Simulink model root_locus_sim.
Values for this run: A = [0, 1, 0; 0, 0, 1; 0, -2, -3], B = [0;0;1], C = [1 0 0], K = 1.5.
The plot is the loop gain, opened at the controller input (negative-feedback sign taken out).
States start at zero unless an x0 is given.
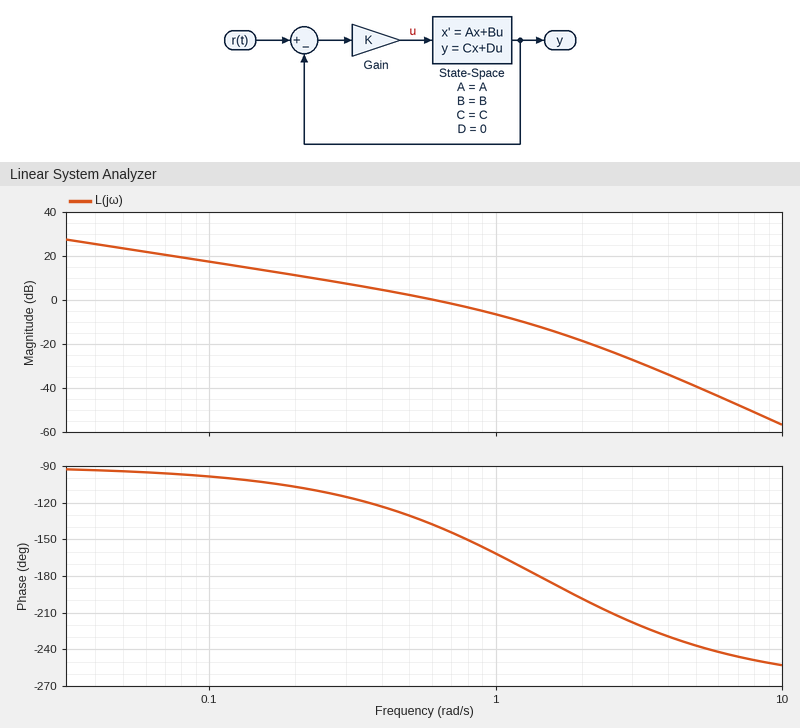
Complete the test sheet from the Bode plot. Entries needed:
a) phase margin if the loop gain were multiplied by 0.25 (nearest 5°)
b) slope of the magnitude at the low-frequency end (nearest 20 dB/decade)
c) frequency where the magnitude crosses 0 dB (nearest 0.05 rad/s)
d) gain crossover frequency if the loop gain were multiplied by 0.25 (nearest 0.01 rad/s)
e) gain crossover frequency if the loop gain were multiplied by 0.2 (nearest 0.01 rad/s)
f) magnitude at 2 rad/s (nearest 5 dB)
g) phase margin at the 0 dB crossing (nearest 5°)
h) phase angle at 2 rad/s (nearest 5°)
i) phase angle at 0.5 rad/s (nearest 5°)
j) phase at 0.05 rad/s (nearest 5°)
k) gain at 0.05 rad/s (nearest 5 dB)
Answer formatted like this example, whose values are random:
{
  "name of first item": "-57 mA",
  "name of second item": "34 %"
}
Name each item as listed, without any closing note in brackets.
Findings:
{
  "phase margin if the loop gain were multiplied by 0.25": "75°",
  "slope of the magnitude at the low-frequency end": "-20 dB/decade",
  "frequency where the magnitude crosses 0 dB": "0.60 rad/s",
  "gain crossover frequency if the loop gain were multiplied by 0.25": "0.18 rad/s",
  "gain crossover frequency if the loop gain were multiplied by 0.2": "0.15 rad/s",
  "magnitude at 2 rad/s": "-20 dB",
  "phase margin at the 0 dB crossing": "40°",
  "phase angle at 2 rad/s": "-200°",
  "phase angle at 0.5 rad/s": "-130°",
  "phase at 0.05 rad/s": "-95°",
  "gain at 0.05 rad/s": "25 dB"
}
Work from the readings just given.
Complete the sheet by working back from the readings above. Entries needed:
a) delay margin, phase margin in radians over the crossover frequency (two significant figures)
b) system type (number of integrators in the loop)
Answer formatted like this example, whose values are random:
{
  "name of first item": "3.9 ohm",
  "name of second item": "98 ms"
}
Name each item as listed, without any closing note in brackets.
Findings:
{
  "delay margin, phase margin in radians over the crossover frequency": "1.2 s",
  "system type": "1"
}
